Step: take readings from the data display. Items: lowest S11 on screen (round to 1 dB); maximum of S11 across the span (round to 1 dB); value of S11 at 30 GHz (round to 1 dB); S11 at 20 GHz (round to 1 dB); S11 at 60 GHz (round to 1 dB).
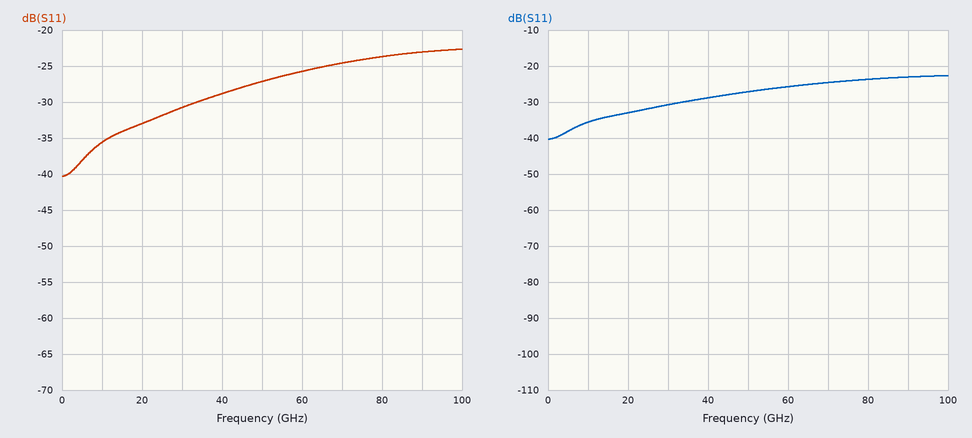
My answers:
-40 dB
-23 dB
-31 dB
-33 dB
-26 dB
